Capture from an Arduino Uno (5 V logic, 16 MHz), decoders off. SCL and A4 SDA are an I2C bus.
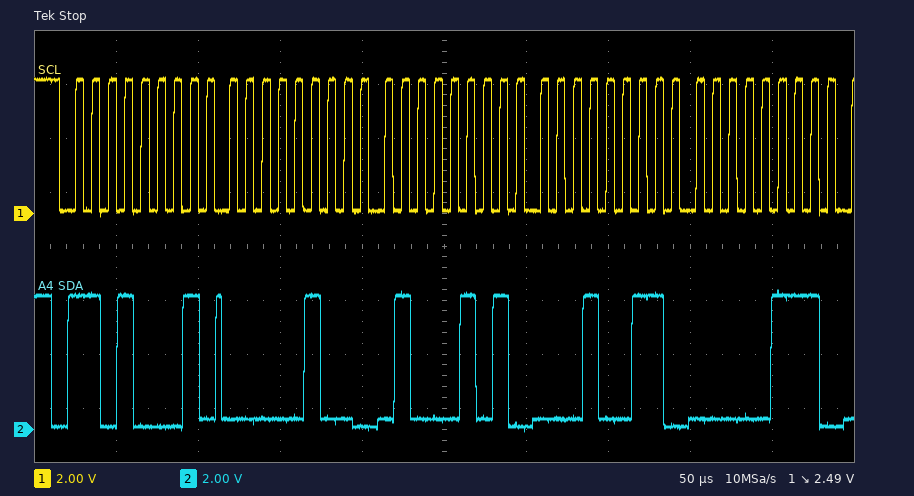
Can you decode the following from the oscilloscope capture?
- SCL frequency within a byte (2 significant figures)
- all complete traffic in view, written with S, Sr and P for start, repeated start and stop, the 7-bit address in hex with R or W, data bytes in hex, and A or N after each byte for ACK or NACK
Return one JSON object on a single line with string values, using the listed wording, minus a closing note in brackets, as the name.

{"SCL frequency within a byte": "100 kHz", "all complete traffic in view, written with S, Sr and P for start, repeated start and stop, the 7-bit address in hex with R or W, data bytes in hex, and A or N after each byte for ACK or NACK": "S 68R A 04 A 45 A 13 A 07 A"}
